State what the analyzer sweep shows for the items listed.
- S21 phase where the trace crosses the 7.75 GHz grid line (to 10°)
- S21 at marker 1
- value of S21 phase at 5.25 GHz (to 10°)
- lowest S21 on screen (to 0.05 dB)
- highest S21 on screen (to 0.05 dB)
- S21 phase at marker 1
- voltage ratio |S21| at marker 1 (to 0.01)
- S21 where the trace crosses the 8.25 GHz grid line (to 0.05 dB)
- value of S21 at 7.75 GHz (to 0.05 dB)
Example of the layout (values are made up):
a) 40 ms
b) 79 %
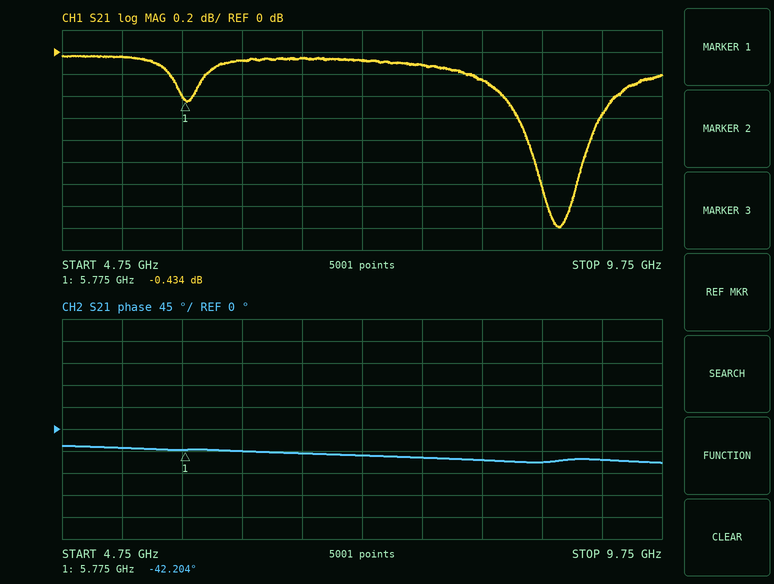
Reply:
a) -60°
b) -0.434 dB
c) -40°
d) -1.60 dB
e) -0.05 dB
f) -42.204°
g) 0.95
h) -0.25 dB
i) -0.10 dB
